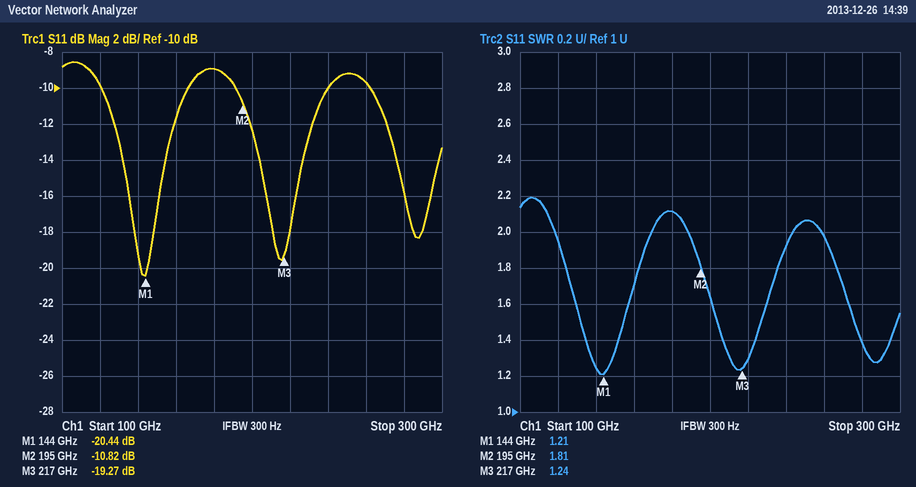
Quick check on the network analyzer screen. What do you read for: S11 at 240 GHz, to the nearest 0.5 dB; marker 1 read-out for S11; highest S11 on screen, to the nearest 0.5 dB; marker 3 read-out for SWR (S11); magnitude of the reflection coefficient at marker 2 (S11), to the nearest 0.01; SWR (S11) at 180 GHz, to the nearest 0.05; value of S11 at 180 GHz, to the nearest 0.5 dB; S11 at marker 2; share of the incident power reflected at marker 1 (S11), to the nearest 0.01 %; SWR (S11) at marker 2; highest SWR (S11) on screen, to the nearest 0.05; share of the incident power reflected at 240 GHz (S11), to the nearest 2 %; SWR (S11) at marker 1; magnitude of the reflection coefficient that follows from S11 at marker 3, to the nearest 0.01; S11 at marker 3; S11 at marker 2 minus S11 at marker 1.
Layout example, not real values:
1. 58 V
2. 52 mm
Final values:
1. -10.0 dB
2. -20.44 dB
3. -8.5 dB
4. 1.24
5. 0.29
6. 2.10
7. -9.0 dB
8. -10.82 dB
9. 0.90 %
10. 1.81
11. 2.20
12. 10 %
13. 1.21
14. 0.11
15. -19.27 dB
16. 9.62 dB
